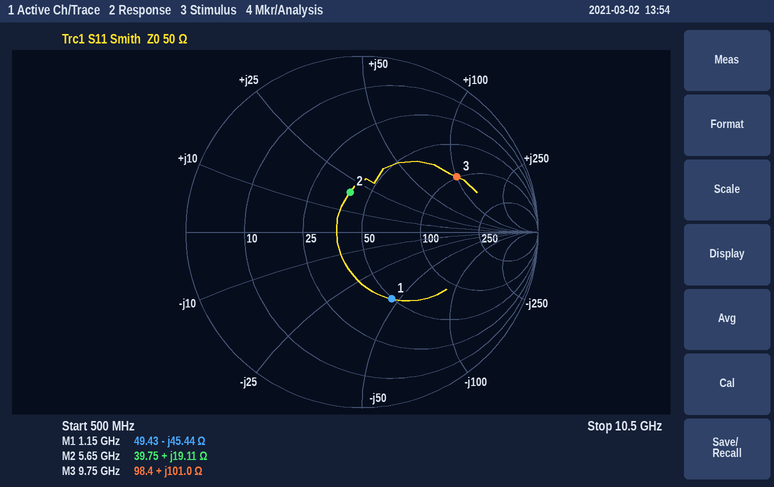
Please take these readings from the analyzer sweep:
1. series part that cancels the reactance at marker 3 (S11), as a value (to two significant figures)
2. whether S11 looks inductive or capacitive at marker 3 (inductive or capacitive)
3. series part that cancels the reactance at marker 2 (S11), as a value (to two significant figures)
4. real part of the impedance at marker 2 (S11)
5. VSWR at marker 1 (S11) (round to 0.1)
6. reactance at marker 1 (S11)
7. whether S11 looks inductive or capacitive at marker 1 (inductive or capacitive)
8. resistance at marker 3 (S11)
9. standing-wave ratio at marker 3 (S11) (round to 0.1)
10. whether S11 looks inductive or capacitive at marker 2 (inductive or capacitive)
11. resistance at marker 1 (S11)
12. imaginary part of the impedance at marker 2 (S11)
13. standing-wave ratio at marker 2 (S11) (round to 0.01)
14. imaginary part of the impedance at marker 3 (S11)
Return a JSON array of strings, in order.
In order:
["160 fF", "inductive", "1.5 pF", "39.75 Ω", "2.4", "-45.44 Ω", "capacitive", "98.4 Ω", "4.3", "inductive", "49.43 Ω", "+19.11 Ω", "1.62", "+101.0 Ω"]
